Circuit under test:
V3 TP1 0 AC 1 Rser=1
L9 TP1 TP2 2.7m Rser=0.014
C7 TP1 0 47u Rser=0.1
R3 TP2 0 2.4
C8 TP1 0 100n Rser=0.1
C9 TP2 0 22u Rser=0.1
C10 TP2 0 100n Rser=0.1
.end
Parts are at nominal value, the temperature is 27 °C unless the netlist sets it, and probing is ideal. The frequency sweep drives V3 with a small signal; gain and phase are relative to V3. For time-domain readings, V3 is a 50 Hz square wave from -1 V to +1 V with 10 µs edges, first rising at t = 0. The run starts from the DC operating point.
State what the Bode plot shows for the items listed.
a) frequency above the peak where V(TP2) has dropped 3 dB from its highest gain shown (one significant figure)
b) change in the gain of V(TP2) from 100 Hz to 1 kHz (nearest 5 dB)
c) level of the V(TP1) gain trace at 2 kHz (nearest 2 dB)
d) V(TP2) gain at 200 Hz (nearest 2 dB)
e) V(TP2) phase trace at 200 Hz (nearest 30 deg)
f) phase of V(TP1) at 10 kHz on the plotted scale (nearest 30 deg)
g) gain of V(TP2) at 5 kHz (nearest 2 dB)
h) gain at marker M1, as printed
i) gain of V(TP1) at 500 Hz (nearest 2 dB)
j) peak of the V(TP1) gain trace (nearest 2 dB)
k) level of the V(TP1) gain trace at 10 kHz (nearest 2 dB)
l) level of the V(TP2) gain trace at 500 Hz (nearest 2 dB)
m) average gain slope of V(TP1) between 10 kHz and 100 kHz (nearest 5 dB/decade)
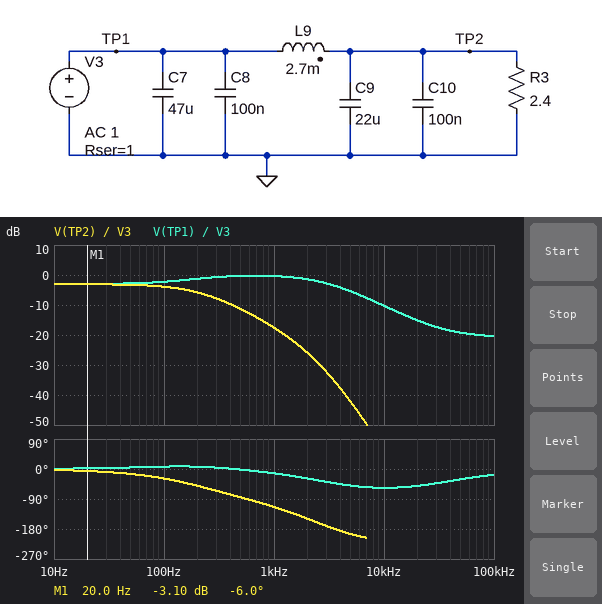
200 Hz
-15 dB
-2 dB
-6 dB
-60 deg
-60 deg
-42 dB
-3.10 dB
0 dB
0 dB
-10 dB
-12 dB
-10 dB/decade
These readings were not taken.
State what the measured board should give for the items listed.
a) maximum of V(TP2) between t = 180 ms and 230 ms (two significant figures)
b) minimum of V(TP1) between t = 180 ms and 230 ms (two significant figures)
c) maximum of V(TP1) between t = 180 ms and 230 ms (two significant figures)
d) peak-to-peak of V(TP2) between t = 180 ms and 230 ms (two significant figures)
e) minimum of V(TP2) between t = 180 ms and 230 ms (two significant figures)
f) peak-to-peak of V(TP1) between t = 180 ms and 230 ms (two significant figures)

700 mV
-1.2 V
1.2 V
1.4 V
-700 mV
2.4 V
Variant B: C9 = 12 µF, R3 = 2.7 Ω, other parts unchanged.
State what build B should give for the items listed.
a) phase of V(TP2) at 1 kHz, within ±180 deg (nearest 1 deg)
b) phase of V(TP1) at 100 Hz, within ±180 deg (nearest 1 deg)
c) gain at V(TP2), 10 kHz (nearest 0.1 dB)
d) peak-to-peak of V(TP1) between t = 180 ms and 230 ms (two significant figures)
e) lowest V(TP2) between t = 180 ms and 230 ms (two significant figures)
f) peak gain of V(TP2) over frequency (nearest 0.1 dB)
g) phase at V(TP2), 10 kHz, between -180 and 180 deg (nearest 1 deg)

-106 deg
6 deg
-53.6 dB
2.3 V
-730 mV
-2.8 dB
153 deg
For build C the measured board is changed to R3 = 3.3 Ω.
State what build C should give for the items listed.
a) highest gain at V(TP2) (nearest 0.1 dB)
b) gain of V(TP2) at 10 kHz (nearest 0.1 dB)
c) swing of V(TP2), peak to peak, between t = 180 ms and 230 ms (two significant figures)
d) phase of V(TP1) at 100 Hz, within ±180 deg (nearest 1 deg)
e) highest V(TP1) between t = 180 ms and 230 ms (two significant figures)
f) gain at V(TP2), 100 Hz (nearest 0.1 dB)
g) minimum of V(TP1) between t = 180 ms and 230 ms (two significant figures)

-2.3 dB
-58.0 dB
1.5 V
4 deg
1.1 V
-2.8 dB
-1.1 V
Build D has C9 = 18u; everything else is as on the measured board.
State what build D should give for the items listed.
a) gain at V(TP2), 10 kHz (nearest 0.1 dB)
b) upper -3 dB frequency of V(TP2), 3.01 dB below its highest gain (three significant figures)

-56.7 dB
212 Hz
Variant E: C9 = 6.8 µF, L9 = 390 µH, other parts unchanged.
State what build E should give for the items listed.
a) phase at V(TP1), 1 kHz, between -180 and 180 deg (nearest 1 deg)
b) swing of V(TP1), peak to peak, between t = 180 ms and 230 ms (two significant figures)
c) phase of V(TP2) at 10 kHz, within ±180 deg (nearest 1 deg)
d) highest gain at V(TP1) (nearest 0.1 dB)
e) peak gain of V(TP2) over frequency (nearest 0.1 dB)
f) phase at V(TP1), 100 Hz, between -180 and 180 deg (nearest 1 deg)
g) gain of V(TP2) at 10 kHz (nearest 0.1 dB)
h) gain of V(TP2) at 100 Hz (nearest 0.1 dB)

-4 deg
1.9 V
172 deg
-1.5 dB
-3.1 dB
0 deg
-33.3 dB
-3.1 dB
